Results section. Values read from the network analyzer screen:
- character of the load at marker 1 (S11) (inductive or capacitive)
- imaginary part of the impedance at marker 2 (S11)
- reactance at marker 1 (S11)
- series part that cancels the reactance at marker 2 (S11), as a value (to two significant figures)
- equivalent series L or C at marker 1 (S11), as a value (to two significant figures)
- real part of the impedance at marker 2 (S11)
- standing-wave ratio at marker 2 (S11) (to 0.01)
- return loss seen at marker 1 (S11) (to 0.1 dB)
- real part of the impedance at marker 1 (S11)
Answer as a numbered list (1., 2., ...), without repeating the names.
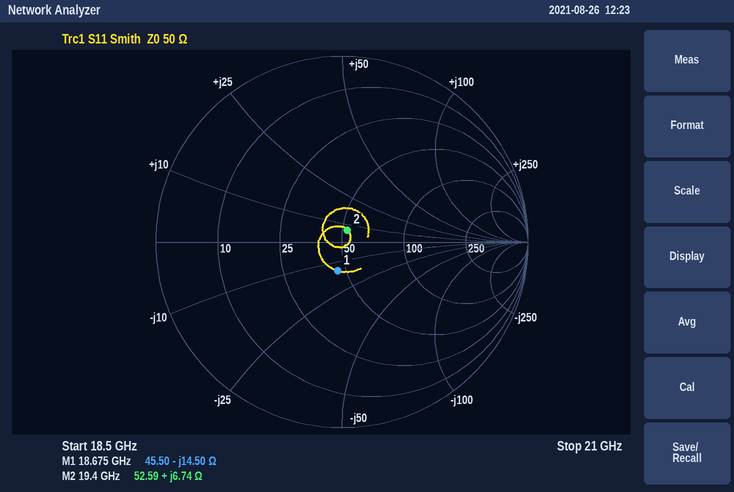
1. capacitive
2. +6.74 Ω
3. -14.50 Ω
4. 1.2 pF
5. 590 fF
6. 52.59 Ω
7. 1.15
8. 16.1 dB
9. 45.50 Ω
